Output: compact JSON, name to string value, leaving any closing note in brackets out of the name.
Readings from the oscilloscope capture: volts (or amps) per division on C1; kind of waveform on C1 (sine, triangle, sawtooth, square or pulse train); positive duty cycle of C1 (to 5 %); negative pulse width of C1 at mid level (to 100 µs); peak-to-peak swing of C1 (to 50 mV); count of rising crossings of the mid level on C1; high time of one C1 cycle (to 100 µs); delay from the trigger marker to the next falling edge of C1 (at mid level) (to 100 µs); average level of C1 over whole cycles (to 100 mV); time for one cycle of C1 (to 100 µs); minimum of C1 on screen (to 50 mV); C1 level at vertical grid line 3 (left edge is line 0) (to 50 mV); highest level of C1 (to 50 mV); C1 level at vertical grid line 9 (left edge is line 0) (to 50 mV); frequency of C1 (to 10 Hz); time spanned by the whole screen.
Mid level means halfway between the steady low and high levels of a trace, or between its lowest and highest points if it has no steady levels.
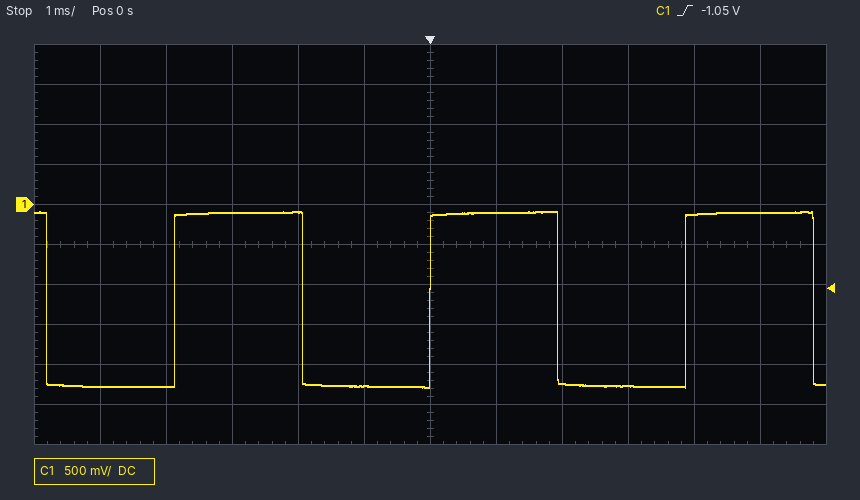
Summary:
{"volts (or amps) per division on C1": "500 mV", "kind of waveform on C1": "square", "positive duty cycle of C1": "50 %", "negative pulse width of C1 at mid level": "1.9 ms", "peak-to-peak swing of C1": "2.20 V", "count of rising crossings of the mid level on C1": "3", "high time of one C1 cycle": "1.9 ms", "delay from the trigger marker to the next falling edge of C1 (at mid level)": "1.9 ms", "average level of C1 over whole cycles": "-1.2 V", "time for one cycle of C1": "3.9 ms", "minimum of C1 on screen": "-2.30 V", "C1 level at vertical grid line 3 (left edge is line 0)": "-100 mV", "highest level of C1": "-100 mV", "C1 level at vertical grid line 9 (left edge is line 0)": "-2.25 V", "frequency of C1": "260 Hz", "time spanned by the whole screen": "12 ms"}
